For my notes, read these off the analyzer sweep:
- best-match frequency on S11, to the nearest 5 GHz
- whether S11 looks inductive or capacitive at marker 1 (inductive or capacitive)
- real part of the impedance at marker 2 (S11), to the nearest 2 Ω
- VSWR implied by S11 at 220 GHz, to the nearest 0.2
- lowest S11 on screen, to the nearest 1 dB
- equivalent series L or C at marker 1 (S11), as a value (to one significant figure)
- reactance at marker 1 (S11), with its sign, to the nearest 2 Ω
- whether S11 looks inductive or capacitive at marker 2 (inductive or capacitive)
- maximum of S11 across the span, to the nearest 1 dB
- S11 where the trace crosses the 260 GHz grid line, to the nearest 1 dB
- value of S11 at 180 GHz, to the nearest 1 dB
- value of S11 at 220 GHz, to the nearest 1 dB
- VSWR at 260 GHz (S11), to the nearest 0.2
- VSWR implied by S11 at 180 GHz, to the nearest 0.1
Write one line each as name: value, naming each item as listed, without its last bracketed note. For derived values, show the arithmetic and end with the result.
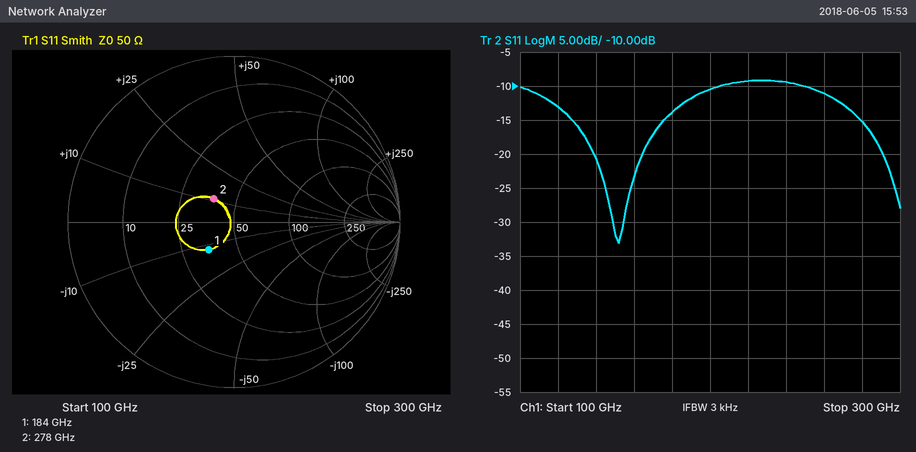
best-match frequency on S11, to the nearest 5 GHz: 150 GHz
whether S11 looks inductive or capacitive at marker 1: capacitive
real part of the impedance at marker 2 (S11), to the nearest 2 Ω: 38 Ω
VSWR implied by S11 at 220 GHz, to the nearest 0.2: |Γ| = 10^(-9/20) = 0.3548; VSWR = (1 + 0.3548)/(1 − 0.3548) ≈ 2.10, so 2.0 to the nearest 0.2
lowest S11 on screen, to the nearest 1 dB: -33 dB
equivalent series L or C at marker 1 (S11), as a value: C = 1/(2π × 184 GHz × 12 Ω) ≈ 72.1 fF, so 70 fF to one significant figure
reactance at marker 1 (S11), with its sign, to the nearest 2 Ω: -12 Ω
whether S11 looks inductive or capacitive at marker 2: inductive
maximum of S11 across the span, to the nearest 1 dB: -9 dB
S11 where the trace crosses the 260 GHz grid line, to the nearest 1 dB: -11 dB
value of S11 at 180 GHz, to the nearest 1 dB: -14 dB
value of S11 at 220 GHz, to the nearest 1 dB: -9 dB
VSWR at 260 GHz (S11), to the nearest 0.2: |Γ| = 10^(-11/20) = 0.2818; VSWR = (1 + 0.2818)/(1 − 0.2818) ≈ 1.8
VSWR implied by S11 at 180 GHz, to the nearest 0.1: |Γ| = 10^(-14/20) = 0.1995; VSWR = (1 + 0.1995)/(1 − 0.1995) ≈ 1.5
